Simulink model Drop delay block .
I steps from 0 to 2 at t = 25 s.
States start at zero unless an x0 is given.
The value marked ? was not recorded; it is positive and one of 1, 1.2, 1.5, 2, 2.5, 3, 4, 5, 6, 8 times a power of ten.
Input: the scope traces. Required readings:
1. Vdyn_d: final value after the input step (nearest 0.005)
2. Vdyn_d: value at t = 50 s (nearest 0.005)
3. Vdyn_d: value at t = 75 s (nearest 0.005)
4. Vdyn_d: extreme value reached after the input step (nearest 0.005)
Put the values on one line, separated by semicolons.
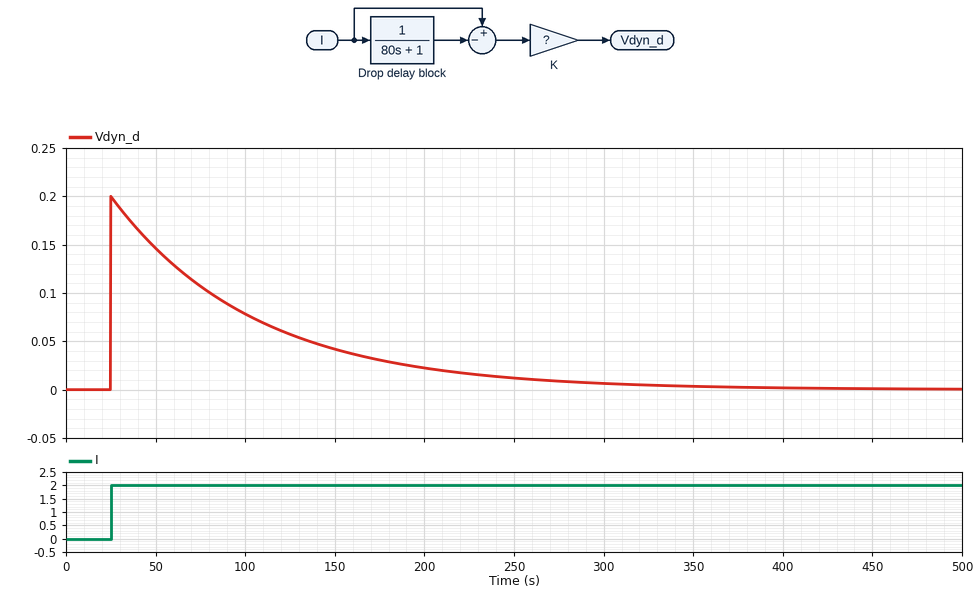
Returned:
0.000; 0.145; 0.105; 0.200
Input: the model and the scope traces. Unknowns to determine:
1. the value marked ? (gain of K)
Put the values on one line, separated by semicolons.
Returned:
0.1
